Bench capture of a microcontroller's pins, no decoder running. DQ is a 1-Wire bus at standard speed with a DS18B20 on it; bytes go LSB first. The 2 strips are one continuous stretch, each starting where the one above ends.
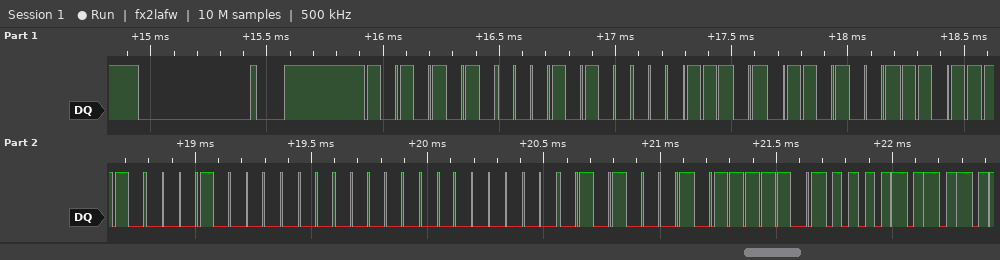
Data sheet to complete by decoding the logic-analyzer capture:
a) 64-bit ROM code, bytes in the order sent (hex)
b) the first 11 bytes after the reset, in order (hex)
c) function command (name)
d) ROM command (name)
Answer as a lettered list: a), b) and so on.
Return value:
a) 28 B8 96 7B 08 00 00 8A
b) 55 28 B8 96 7B 08 00 00 8A BE 50
c) Read Scratchpad
d) Match ROM
